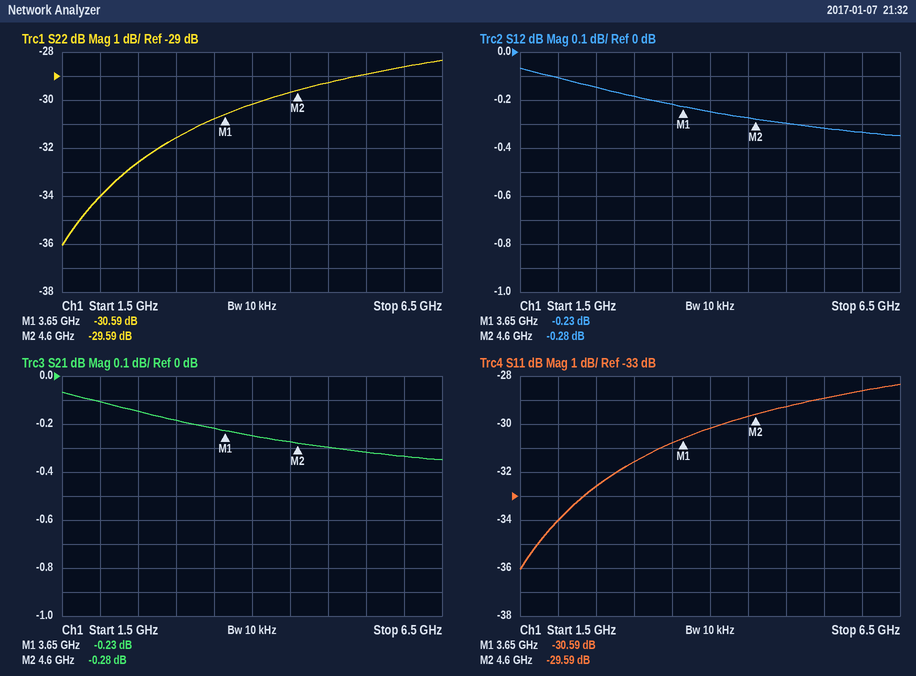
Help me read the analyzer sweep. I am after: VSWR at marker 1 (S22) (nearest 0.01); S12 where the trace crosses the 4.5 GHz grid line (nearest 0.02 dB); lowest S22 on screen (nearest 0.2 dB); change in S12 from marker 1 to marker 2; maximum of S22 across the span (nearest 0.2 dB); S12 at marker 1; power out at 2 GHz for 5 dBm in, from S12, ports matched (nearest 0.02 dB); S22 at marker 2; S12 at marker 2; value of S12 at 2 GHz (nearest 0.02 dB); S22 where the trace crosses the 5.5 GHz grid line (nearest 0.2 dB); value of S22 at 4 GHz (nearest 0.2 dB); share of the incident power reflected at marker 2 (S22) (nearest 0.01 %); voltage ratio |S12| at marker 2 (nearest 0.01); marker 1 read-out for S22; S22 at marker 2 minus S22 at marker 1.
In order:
1.06
-0.28 dB
-36.0 dB
-0.05 dB
-28.4 dB
-0.23 dB
4.90 dBm
-29.59 dB
-0.28 dB
-0.10 dB
-29.0 dB
-30.2 dB
0.11 %
0.97
-30.59 dB
1.00 dB
